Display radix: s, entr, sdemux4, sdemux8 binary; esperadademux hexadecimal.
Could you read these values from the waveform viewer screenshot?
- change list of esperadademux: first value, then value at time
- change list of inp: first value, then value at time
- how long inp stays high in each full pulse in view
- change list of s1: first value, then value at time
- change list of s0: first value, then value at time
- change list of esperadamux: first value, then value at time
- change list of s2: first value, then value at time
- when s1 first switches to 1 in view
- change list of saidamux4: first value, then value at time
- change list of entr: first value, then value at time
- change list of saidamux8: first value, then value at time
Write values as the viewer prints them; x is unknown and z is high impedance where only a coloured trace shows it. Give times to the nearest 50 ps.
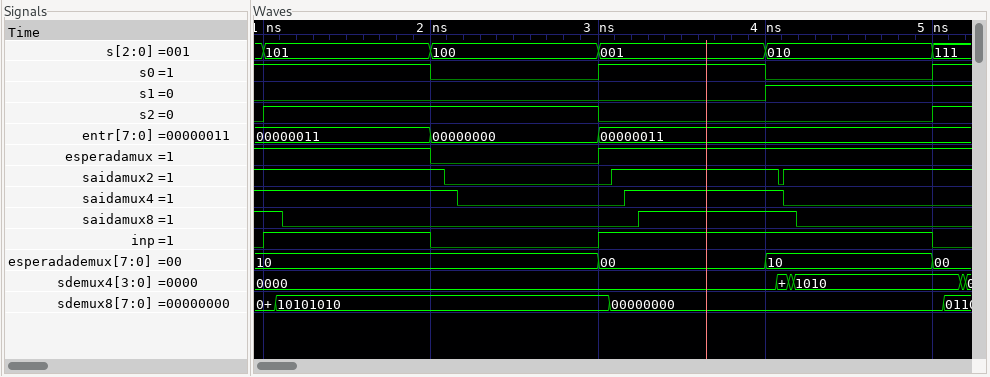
10, 00 at 3000 ps, 10 at 4000 ps, 00 at 5000 ps
0, 1 at 1000 ps, 0 at 2000 ps, 1 at 3000 ps, 0 at 5000 ps
1000 ps, 2000 ps
0, 1 at 4000 ps
1, 0 at 2000 ps, 1 at 3000 ps, 0 at 4000 ps, 1 at 5000 ps
1, 0 at 2000 ps, 1 at 3000 ps
0, 1 at 1000 ps, 0 at 3000 ps, 1 at 5000 ps
4000 ps
1, 0 at 2150 ps, 1 at 3150 ps, 0 at 4100 ps
00000011, 00000000 at 2000 ps, 00000011 at 3000 ps
1, 0 at 1100 ps, 1 at 3250 ps, 0 at 4200 ps
